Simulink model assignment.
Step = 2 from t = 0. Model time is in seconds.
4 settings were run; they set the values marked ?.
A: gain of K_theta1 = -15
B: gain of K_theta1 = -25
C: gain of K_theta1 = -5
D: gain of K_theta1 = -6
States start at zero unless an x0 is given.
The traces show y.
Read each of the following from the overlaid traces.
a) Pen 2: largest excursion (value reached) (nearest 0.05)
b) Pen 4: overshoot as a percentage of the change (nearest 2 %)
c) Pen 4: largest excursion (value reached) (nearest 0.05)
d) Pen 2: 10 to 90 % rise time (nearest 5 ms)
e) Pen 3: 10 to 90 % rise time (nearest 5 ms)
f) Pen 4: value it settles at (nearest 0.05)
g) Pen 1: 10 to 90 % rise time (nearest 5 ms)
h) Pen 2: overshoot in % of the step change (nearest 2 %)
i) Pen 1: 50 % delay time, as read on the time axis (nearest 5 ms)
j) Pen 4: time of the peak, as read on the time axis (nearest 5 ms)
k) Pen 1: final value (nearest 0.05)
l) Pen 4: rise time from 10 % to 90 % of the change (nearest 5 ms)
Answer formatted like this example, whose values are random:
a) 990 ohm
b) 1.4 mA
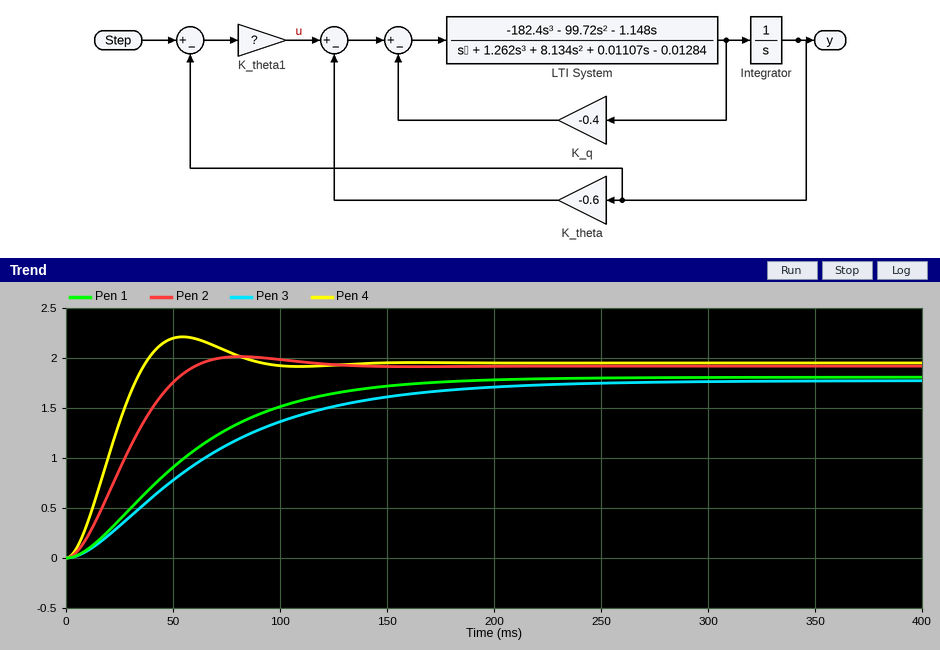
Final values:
a) 2.00
b) 14 %
c) 2.20
d) 40 ms
e) 130 ms
f) 1.95
g) 105 ms
h) 4 %
i) 50 ms
j) 55 ms
k) 1.80
l) 25 ms
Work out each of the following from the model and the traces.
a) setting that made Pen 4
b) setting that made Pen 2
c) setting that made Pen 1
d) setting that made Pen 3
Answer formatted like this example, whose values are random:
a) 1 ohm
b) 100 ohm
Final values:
a) B
b) A
c) D
d) C
